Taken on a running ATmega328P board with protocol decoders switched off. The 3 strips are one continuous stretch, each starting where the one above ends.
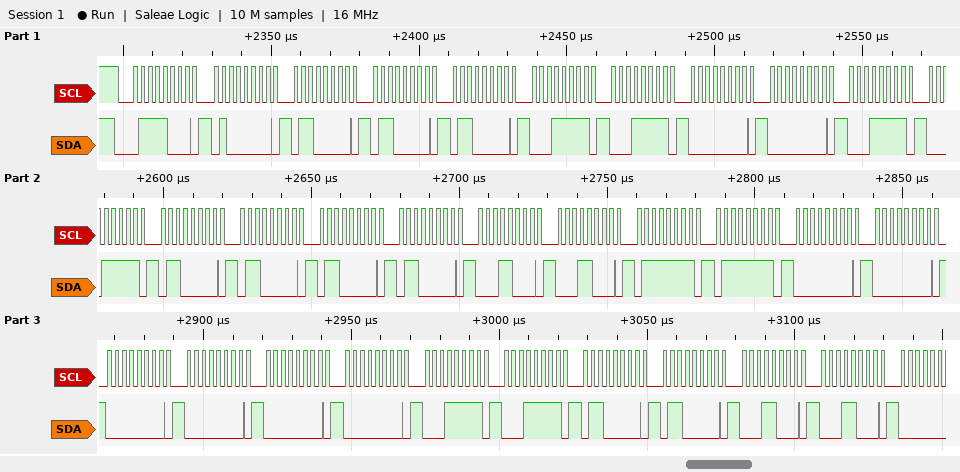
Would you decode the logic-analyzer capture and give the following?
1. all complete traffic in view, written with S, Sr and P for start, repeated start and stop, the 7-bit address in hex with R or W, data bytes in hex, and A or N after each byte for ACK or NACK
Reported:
S 3CW A 40 A 60 A 60 A 60 A 1F A 1F A 00 A 00 A 1F A 1F A 60 A 60 A 60 A 60 A 18 A 18 A 7F A 7F A 00 A 00 A 00 A 00 A 00 A 00 A 1F A 1F A 60 A 60 A 18 A 18 A
